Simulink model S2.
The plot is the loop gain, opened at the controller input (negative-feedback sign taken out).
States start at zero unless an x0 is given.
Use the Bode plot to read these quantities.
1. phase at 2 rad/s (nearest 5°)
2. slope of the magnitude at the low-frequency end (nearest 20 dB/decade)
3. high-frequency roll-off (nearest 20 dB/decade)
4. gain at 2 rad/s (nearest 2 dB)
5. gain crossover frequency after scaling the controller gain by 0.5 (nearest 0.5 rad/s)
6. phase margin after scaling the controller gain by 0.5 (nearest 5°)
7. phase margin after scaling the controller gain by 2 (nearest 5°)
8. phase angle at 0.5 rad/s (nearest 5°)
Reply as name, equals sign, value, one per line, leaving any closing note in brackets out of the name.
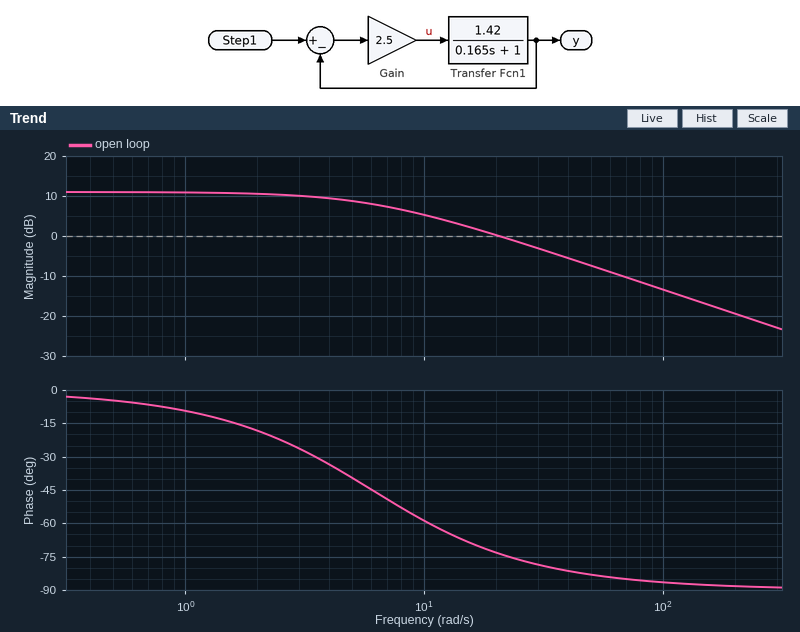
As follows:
phase at 2 rad/s = -20°
slope of the magnitude at the low-frequency end = 0 dB/decade
high-frequency roll-off = -20 dB/decade
gain at 2 rad/s = 10 dB
gain crossover frequency after scaling the controller gain by 0.5 = 9.0 rad/s
phase margin after scaling the controller gain by 0.5 = 125°
phase margin after scaling the controller gain by 2 = 100°
phase angle at 0.5 rad/s = -5°
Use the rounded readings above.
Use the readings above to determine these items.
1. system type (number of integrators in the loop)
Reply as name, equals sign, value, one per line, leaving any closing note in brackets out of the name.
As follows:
system type = 0
